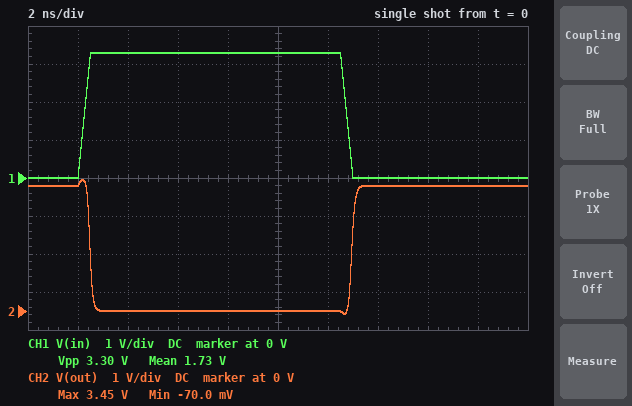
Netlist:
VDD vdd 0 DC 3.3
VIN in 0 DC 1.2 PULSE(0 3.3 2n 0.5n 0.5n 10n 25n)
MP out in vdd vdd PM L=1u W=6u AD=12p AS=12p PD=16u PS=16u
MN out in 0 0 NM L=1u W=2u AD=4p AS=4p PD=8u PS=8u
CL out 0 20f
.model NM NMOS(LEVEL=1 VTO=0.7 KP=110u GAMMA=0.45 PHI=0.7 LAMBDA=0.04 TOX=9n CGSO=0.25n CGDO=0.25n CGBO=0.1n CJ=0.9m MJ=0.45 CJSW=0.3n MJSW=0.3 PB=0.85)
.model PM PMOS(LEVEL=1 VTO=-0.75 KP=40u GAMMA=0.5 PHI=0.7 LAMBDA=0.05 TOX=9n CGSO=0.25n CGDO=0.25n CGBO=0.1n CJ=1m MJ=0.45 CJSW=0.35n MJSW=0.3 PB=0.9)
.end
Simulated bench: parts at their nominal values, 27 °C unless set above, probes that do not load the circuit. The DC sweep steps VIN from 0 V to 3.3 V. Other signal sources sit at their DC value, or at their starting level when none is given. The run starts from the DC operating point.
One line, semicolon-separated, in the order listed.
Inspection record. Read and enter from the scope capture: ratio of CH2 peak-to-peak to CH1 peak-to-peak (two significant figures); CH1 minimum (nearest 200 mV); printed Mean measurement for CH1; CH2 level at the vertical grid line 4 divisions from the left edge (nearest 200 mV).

1.1; 0 V; 1.73 V; 0 V
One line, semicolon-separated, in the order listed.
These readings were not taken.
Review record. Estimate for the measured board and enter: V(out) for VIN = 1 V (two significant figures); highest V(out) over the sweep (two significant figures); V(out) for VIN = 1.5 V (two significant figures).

3.3 V; 3.3 V; 2.9 V
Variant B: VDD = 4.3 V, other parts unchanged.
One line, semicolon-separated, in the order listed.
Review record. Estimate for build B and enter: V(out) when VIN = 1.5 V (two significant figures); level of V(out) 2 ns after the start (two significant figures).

4.1 V; 4.3 V
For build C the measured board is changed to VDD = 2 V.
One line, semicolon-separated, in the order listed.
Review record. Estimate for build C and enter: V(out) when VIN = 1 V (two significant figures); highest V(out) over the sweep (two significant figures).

170 mV; 2.0 V
